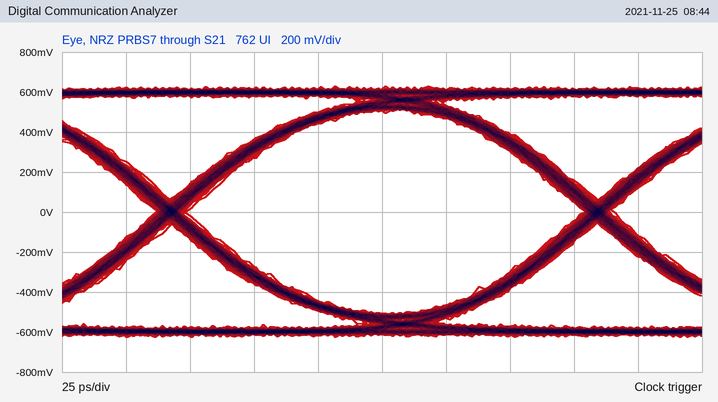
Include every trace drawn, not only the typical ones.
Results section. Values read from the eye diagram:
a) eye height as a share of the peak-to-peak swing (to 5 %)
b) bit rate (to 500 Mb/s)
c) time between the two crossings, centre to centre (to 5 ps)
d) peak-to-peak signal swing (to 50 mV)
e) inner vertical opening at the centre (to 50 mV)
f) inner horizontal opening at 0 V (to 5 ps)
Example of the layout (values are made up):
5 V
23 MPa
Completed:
80 %
6.0 Gb/s
165 ps
1.25 V
1.00 V
155 ps
